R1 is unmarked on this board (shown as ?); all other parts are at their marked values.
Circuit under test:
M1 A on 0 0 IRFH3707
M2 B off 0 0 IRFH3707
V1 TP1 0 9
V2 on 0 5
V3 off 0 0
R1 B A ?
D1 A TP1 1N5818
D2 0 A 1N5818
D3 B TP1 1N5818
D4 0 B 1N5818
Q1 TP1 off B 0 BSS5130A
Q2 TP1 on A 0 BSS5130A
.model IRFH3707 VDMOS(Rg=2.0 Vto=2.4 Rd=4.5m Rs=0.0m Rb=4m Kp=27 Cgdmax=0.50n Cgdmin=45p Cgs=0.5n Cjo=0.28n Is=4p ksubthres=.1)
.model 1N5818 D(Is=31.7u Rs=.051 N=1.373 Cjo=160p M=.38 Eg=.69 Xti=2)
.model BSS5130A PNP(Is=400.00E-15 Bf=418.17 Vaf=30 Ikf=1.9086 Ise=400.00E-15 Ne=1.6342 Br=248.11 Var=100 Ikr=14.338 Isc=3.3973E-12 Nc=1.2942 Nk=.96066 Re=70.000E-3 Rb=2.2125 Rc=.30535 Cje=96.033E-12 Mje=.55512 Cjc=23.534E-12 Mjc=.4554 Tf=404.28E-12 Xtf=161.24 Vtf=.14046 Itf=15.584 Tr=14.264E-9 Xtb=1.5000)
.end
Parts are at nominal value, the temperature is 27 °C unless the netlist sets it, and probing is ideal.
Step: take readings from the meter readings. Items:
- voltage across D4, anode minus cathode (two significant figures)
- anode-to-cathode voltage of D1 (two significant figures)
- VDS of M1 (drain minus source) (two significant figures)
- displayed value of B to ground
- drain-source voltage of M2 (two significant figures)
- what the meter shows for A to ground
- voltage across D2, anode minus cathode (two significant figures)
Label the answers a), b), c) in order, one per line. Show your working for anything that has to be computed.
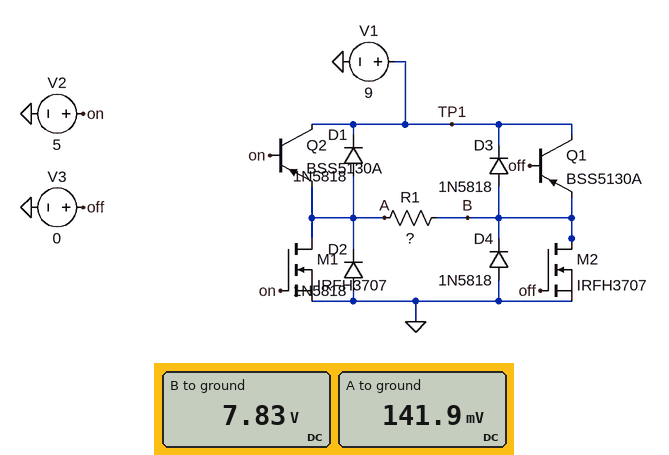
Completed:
a) 0 V - 7.83 V = -7.8 V
b) 141.9 mV - 9 V = -8.9 V
c) 141.9 mV = 140 mV
d) 7.83 V
e) 7.83 V = 7.8 V
f) 141.9 mV
g) 0 V - 141.9 mV = -140 mV
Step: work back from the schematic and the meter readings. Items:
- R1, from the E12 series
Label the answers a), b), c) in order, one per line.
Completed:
a) 15 Ω
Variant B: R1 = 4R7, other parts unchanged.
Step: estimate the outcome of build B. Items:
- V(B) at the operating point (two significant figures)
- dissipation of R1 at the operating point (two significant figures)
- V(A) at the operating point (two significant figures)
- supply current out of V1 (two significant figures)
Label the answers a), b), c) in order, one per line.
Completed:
a) 7.5 V
b) 11 W
c) 160 mV
d) 12 A
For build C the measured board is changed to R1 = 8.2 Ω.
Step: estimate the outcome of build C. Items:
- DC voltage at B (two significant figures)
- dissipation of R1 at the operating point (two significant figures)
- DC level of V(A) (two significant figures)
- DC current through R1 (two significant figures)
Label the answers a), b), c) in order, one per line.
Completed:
a) 7.7 V
b) 6.9 W
c) 150 mV
d) 920 mA
